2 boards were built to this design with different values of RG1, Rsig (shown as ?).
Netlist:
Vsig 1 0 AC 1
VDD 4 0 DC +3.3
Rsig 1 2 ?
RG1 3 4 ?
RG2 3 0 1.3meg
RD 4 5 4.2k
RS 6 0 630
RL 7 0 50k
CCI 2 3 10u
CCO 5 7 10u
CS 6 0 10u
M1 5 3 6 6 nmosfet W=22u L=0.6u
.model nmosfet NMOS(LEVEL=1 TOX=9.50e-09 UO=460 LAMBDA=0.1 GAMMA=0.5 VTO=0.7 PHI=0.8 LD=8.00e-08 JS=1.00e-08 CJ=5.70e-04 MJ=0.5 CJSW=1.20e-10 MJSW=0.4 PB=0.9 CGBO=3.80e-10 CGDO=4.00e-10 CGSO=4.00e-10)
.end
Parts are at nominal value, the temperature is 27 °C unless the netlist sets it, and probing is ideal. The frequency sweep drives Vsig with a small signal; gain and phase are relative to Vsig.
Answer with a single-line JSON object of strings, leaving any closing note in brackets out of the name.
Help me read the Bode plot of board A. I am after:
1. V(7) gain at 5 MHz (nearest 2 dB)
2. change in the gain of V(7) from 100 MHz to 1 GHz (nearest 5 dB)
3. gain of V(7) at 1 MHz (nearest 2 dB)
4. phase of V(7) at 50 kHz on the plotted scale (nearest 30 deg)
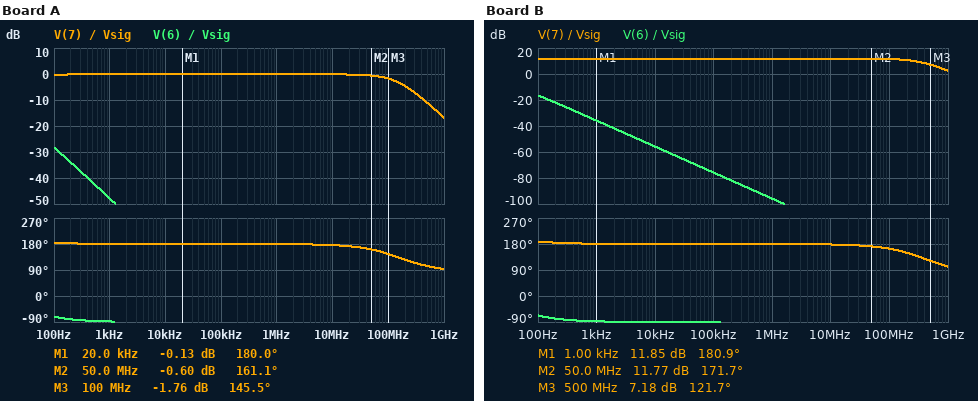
{"V(7) gain at 5 MHz": "0 dB", "change in the gain of V(7) from 100 MHz to 1 GHz": "-15 dB", "gain of V(7) at 1 MHz": "0 dB", "phase of V(7) at 50 kHz on the plotted scale": "180 deg"}
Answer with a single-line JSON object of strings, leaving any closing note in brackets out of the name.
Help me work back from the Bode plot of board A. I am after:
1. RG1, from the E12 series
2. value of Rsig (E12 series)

{"RG1, from the E12 series": "1.5 MΩ", "value of Rsig": "15 kΩ"}
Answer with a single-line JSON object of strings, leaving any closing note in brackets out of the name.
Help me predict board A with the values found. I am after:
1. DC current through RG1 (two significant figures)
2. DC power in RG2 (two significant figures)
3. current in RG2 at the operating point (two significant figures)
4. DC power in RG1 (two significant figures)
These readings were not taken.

{"DC current through RG1": "1.2 µA", "DC power in RG2": "1.8 µW", "current in RG2 at the operating point": "1.2 µA", "DC power in RG1": "2.1 µW"}
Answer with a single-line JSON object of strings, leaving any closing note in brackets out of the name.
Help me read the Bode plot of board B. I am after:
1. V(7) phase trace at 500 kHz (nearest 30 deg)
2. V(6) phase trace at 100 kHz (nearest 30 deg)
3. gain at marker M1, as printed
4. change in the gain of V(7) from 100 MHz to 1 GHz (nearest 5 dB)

{"V(7) phase trace at 500 kHz": "180 deg", "V(6) phase trace at 100 kHz": "-90 deg", "gain at marker M1, as printed": "11.85 dB", "change in the gain of V(7) from 100 MHz to 1 GHz": "-10 dB"}
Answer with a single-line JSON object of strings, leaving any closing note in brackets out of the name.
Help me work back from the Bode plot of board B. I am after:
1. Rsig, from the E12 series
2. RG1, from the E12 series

{"Rsig, from the E12 series": "5.6 kΩ", "RG1, from the E12 series": "3.9 MΩ"}
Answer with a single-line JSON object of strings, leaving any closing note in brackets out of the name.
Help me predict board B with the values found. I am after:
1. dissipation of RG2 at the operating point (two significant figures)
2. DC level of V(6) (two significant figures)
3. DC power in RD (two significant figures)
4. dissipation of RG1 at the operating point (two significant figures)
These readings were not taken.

{"dissipation of RG2 at the operating point": "520 nW", "DC level of V(6)": "31 mV", "DC power in RD": "9.9 µW", "dissipation of RG1 at the operating point": "1.6 µW"}
